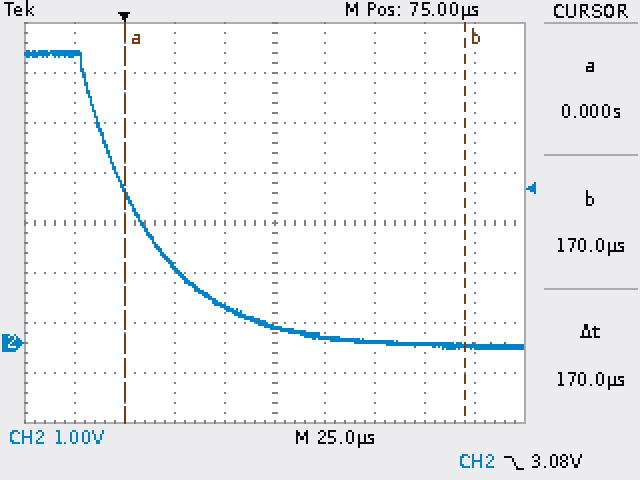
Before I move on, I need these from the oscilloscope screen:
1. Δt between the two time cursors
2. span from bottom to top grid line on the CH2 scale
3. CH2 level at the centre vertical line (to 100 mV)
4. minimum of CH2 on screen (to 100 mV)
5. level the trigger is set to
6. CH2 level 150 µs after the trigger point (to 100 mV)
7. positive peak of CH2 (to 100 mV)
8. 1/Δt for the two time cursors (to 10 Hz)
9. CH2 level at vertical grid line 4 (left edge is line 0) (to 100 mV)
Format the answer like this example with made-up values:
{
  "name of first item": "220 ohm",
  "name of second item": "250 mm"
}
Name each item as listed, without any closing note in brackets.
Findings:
{
  "Δt between the two time cursors": "170 µs",
  "span from bottom to top grid line on the CH2 scale": "8 V",
  "CH2 level at the centre vertical line": "300 mV",
  "minimum of CH2 on screen": "-100 mV",
  "level the trigger is set to": "3.08 V",
  "CH2 level 150 µs after the trigger point": "0.0 V",
  "positive peak of CH2": "5.8 V",
  "1/Δt for the two time cursors": "5.88 kHz",
  "CH2 level at vertical grid line 4 (left edge is line 0)": "700 mV"
}
